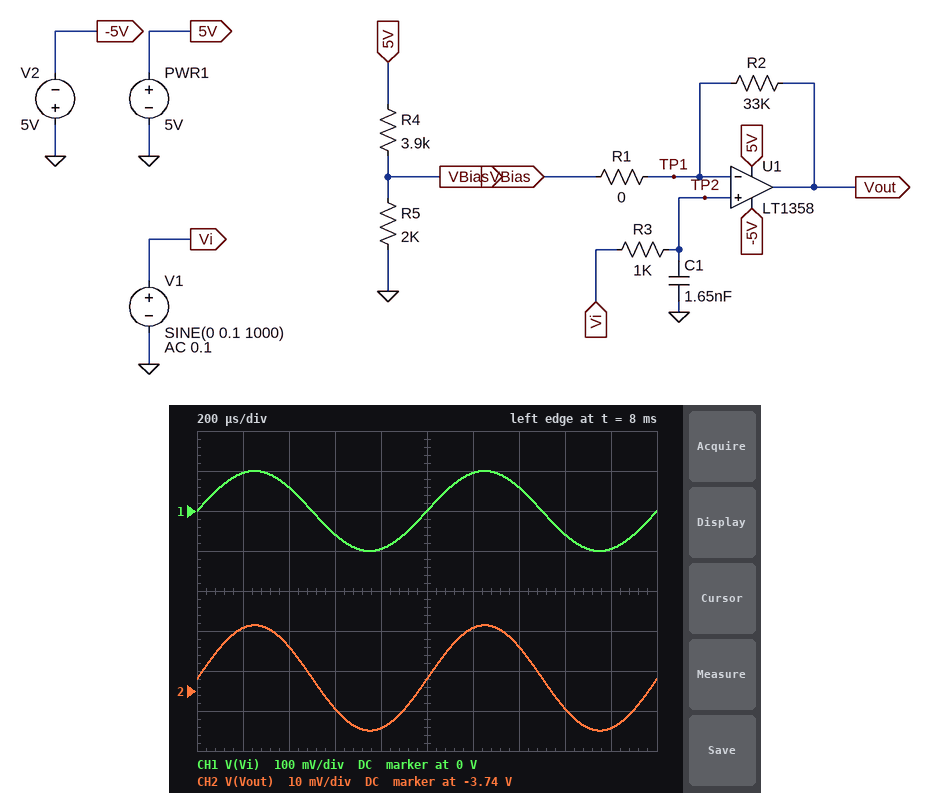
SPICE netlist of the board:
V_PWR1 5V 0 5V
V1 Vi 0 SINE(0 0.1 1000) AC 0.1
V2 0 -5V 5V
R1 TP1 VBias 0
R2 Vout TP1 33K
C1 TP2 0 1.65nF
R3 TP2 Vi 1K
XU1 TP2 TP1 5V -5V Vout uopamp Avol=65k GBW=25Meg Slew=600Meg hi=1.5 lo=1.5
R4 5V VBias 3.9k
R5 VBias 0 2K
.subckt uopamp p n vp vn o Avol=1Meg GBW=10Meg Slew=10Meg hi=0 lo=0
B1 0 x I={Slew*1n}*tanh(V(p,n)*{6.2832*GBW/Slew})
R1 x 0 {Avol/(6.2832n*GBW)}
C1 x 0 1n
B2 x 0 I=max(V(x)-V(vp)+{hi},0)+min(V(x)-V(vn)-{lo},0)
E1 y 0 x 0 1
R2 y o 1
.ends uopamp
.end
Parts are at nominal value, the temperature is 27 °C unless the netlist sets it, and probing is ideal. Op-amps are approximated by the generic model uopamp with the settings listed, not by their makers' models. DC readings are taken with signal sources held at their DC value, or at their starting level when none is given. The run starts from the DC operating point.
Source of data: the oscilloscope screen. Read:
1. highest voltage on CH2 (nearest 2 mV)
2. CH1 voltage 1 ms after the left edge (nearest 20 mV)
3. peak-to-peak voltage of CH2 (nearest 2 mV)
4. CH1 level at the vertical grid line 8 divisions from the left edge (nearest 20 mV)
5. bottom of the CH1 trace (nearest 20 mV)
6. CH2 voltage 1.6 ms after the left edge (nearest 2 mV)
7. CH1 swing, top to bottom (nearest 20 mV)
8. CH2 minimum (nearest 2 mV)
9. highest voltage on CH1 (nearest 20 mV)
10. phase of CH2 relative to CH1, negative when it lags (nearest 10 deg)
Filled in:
-3.724 V
0 V
26 mV
-60 mV
-100 mV
-3.744 V
200 mV
-3.750 V
100 mV
0 deg
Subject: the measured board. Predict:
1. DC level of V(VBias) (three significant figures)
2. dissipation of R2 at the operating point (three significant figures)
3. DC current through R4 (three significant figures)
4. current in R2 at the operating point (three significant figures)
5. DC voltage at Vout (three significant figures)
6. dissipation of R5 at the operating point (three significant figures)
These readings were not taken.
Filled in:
1.60 V
862 µW
873 µA
162 µA
-3.74 V
1.27 mW
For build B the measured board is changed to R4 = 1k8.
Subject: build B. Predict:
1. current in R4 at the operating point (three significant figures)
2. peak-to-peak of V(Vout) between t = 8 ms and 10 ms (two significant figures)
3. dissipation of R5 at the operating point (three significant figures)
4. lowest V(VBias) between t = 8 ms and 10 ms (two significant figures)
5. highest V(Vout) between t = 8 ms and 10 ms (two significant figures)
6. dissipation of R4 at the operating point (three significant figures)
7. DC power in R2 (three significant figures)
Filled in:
1.26 mA
20 mV
3.71 mW
2.7 V
-3.9 V
2.88 mW
1.32 mW
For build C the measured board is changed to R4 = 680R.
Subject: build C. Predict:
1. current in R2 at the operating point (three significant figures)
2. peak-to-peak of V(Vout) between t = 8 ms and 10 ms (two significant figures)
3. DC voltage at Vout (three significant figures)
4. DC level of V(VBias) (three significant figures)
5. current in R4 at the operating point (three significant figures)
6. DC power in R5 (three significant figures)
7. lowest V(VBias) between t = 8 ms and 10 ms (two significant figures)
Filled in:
232 µA
14 mV
-3.95 V
3.70 V
1.91 mA
6.86 mW
3.7 V
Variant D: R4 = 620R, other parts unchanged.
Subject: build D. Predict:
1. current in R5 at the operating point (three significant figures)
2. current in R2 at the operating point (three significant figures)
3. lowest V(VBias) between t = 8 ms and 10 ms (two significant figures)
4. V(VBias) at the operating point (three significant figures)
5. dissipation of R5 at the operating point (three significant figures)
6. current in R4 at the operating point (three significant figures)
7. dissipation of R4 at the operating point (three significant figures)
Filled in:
2.03 mA
244 µA
4.1 V
4.07 V
8.27 mW
1.50 mA
1.40 mW
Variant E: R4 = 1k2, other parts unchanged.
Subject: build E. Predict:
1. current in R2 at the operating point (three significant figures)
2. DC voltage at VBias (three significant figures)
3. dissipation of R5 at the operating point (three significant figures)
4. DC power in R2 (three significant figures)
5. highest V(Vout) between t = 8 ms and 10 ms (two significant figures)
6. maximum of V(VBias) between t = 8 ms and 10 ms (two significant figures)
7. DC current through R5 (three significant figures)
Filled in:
201 µA
2.76 V
3.82 mW
1.33 mW
-3.9 V
2.8 V
1.38 mA
